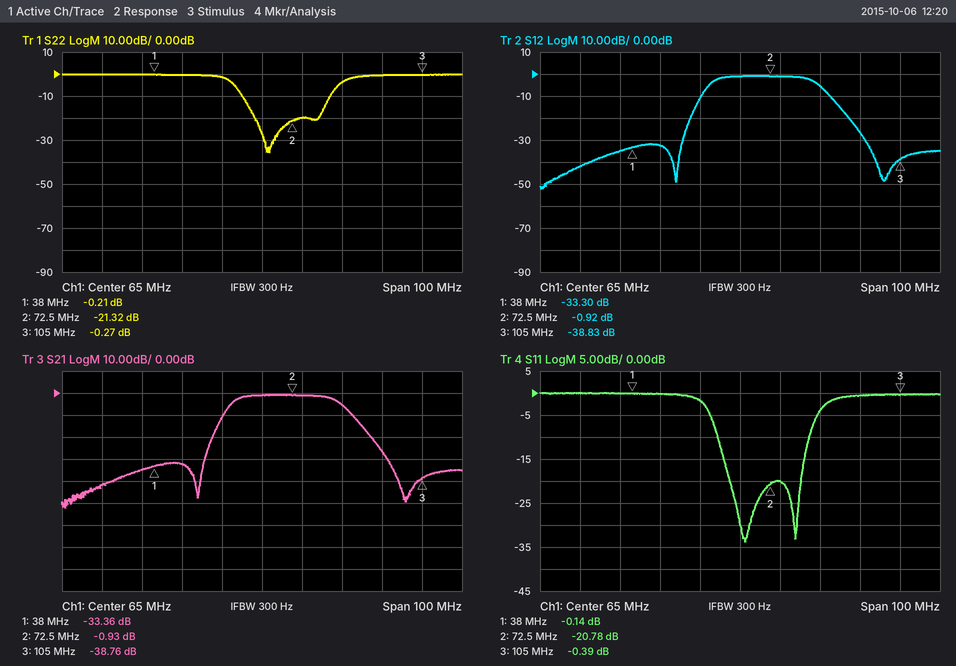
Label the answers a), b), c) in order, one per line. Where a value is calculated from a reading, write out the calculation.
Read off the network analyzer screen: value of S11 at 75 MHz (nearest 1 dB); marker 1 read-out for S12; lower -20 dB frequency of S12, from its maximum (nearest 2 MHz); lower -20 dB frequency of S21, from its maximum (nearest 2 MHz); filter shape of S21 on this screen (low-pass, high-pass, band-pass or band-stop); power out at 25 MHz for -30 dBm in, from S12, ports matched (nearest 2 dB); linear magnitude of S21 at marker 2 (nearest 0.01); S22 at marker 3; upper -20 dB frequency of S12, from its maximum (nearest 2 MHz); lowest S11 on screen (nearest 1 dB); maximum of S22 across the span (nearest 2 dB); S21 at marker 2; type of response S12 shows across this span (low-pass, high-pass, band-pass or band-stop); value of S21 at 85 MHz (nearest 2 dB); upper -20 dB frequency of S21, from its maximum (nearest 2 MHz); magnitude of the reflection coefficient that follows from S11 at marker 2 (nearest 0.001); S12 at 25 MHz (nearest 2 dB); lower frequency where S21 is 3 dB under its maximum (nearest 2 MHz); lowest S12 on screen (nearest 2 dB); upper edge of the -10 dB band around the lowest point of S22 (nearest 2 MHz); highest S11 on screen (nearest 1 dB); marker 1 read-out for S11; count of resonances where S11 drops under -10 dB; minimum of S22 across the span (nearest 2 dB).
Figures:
a) -20 dB
b) -33.30 dB
c) 52 MHz
d) 52 MHz
e) band-pass
f) -30 dBm + (-42 dB) = -72 dBm
g) 10^(-0.93/20) ≈ 0.90
h) -0.27 dB
i) 92 MHz
j) -34 dB
k) 0 dB
l) -0.93 dB
m) band-pass
n) -6 dB
o) 92 MHz
p) 10^(-20.78/20) ≈ 0.091
q) -42 dB
r) 58 MHz
s) -52 dB
t) 82 MHz
u) 0 dB
v) -0.14 dB
w) 2
x) -36 dB
